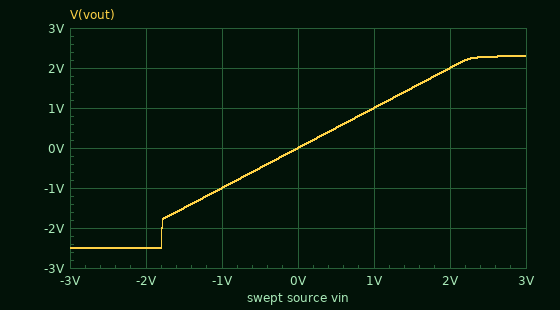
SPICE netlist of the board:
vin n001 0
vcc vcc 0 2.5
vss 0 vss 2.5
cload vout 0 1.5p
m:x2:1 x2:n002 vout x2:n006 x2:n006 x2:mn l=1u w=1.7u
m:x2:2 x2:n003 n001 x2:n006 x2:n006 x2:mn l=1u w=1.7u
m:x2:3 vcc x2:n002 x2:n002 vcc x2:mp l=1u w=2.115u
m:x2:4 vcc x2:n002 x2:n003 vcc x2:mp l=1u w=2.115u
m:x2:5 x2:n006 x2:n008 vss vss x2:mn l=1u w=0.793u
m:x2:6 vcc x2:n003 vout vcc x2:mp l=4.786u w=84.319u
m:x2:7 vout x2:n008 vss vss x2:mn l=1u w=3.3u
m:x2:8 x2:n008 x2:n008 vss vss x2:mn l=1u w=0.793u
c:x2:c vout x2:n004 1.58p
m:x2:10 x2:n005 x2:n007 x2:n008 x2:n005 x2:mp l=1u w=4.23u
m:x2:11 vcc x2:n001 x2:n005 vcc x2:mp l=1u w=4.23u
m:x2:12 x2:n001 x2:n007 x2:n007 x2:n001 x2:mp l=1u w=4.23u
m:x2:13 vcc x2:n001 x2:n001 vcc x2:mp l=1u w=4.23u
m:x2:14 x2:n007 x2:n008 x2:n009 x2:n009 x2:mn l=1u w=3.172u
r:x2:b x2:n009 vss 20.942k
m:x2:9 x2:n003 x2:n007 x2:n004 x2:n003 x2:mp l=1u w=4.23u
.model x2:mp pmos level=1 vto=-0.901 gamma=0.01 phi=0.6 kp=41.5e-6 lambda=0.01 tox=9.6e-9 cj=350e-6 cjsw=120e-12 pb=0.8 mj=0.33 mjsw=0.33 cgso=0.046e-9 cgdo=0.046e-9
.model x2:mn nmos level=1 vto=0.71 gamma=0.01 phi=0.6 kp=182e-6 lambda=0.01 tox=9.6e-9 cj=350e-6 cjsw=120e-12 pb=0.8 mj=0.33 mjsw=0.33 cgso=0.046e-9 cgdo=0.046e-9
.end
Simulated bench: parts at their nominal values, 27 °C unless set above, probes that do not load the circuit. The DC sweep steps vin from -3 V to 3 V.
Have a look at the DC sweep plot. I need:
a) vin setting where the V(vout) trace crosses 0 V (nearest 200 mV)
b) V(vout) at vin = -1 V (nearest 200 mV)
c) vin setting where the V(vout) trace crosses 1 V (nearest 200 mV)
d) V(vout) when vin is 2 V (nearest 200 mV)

0 V
-1.0 V
1.0 V
2.0 V
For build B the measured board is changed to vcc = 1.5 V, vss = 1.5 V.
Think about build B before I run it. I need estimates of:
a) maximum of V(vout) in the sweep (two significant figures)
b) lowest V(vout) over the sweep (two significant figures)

1.3 V
-1.5 V
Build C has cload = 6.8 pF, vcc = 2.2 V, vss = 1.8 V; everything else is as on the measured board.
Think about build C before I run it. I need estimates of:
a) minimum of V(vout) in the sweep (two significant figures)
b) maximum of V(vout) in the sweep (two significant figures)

-1.8 V
2.0 V
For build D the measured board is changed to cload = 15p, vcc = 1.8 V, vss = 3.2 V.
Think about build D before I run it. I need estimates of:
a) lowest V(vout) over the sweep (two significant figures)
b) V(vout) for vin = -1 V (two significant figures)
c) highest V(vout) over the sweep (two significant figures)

-3.2 V
-1.0 V
1.6 V
